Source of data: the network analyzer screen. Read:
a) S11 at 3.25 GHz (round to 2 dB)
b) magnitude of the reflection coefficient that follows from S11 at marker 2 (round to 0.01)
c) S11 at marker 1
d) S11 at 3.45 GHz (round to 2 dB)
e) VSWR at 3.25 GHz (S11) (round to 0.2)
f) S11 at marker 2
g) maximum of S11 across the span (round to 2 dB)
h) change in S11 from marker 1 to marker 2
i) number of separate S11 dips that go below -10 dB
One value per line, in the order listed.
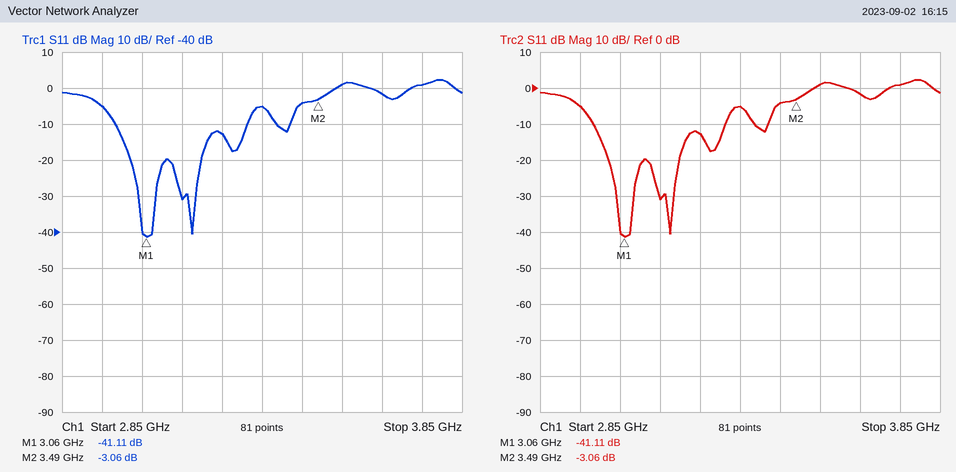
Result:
-12 dB
0.70
-41.11 dB
-4 dB
1.6
-3.06 dB
2 dB
38.05 dB
4
